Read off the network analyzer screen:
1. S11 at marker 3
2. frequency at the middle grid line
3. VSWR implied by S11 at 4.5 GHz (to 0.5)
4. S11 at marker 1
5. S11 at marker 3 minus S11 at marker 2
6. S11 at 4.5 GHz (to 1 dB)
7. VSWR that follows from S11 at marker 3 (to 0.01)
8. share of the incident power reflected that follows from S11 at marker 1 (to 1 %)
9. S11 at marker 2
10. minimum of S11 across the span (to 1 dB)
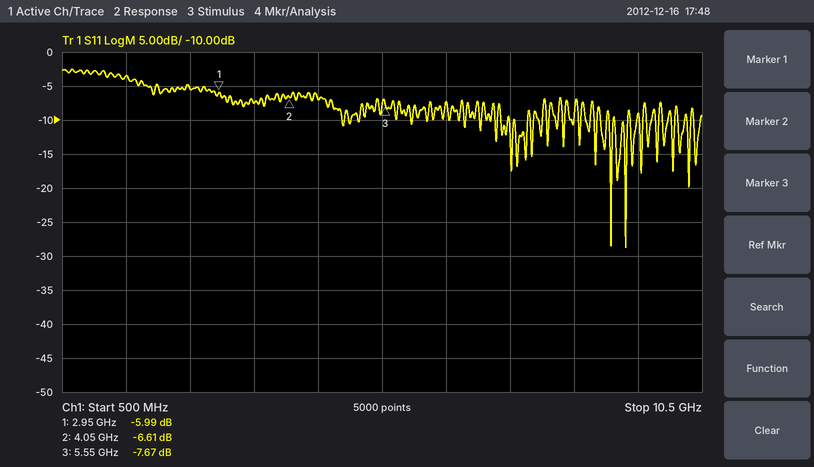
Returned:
-7.67 dB
5.5 GHz
2.5
-5.99 dB
-1.06 dB
-7 dB
2.41
25 %
-6.61 dB
-29 dB
